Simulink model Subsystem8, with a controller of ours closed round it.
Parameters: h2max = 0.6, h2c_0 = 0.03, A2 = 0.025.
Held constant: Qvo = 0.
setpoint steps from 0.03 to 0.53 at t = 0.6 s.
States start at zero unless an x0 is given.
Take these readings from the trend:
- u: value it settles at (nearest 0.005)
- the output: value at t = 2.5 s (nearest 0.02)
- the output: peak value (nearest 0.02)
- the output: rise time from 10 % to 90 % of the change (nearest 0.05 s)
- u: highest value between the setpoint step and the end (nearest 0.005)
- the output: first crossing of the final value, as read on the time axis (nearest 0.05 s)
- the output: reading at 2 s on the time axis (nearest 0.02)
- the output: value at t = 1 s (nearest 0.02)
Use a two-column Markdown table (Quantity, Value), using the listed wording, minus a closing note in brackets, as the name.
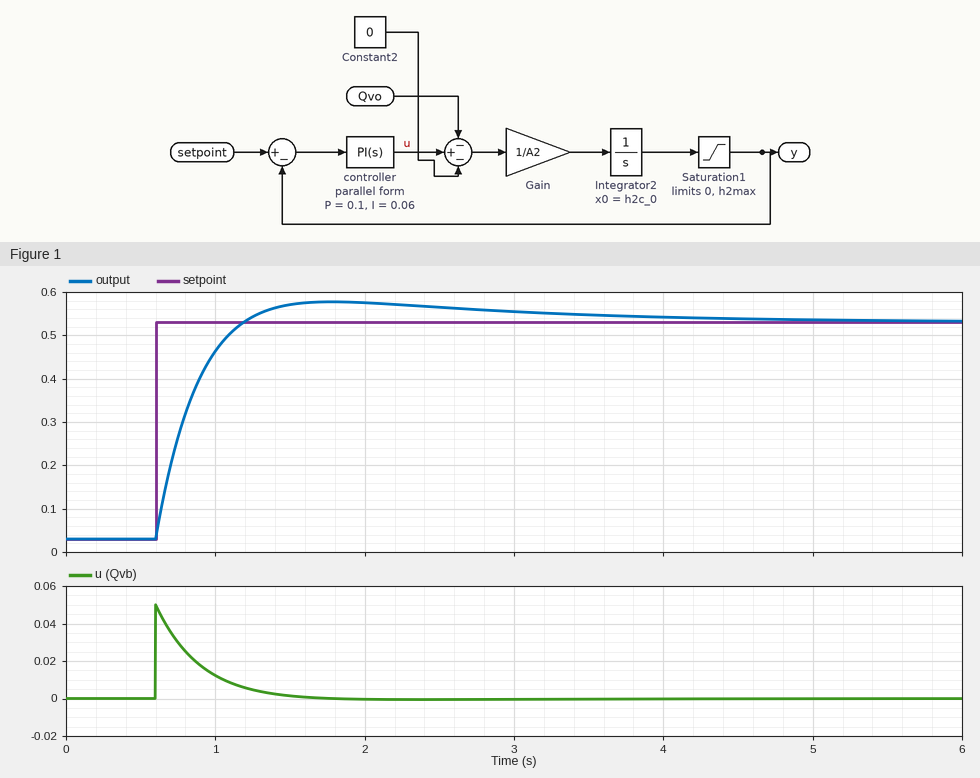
| Quantity | Value |
|---|---|
| u: value it settles at | 0.000 |
| the output: value at t = 2.5 s | 0.56 |
| the output: peak value | 0.58 |
| the output: rise time from 10 % to 90 % of the change | 0.40 s |
| u: highest value between the setpoint step and the end | 0.050 |
| the output: first crossing of the final value, as read on the time axis | 1.20 s |
| the output: reading at 2 s on the time axis | 0.58 |
| the output: value at t = 1 s | 0.46 |
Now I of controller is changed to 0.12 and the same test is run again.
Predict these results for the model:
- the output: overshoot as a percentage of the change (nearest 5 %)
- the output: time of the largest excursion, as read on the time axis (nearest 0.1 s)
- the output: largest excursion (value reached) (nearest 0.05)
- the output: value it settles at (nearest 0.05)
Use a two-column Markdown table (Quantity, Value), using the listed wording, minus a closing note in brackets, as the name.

| Quantity | Value |
|---|---|
| the output: overshoot as a percentage of the change | 15 % |
| the output: time of the largest excursion, as read on the time axis | 1.4 s |
| the output: largest excursion (value reached) | 0.60 |
| the output: value it settles at | 0.55 |
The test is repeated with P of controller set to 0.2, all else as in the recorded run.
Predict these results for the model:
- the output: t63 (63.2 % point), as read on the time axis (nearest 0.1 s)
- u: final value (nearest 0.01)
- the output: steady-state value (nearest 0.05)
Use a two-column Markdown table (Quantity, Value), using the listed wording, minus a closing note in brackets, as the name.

| Quantity | Value |
|---|---|
| the output: t63 (63.2 % point), as read on the time axis | 0.7 s |
| u: final value | 0.00 |
| the output: steady-state value | 0.55 |
